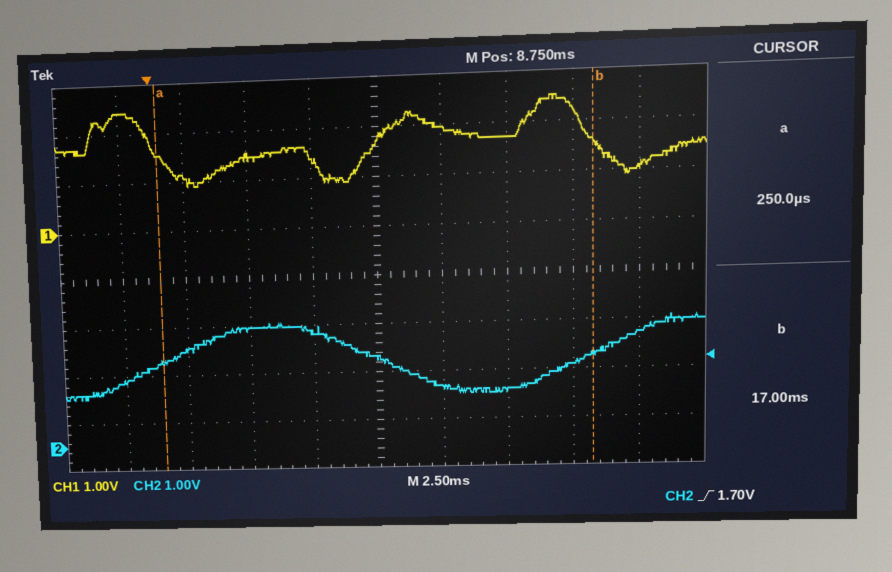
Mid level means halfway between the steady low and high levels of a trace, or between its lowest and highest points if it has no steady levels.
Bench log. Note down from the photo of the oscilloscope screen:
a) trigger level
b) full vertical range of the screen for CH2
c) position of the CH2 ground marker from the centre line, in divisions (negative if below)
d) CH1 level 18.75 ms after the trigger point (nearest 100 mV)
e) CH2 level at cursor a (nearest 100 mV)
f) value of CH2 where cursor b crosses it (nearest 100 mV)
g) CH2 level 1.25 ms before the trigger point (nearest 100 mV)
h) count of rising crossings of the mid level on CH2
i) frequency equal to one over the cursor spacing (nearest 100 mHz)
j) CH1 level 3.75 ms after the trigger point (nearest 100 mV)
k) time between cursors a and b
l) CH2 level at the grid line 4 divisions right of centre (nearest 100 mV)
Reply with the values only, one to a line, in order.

1.70 V
8 V
-3.5 div
1.1 V
1.8 V
1.8 V
1.4 V
2
59.7 Hz
1.5 V
16.75 ms
2.2 V
